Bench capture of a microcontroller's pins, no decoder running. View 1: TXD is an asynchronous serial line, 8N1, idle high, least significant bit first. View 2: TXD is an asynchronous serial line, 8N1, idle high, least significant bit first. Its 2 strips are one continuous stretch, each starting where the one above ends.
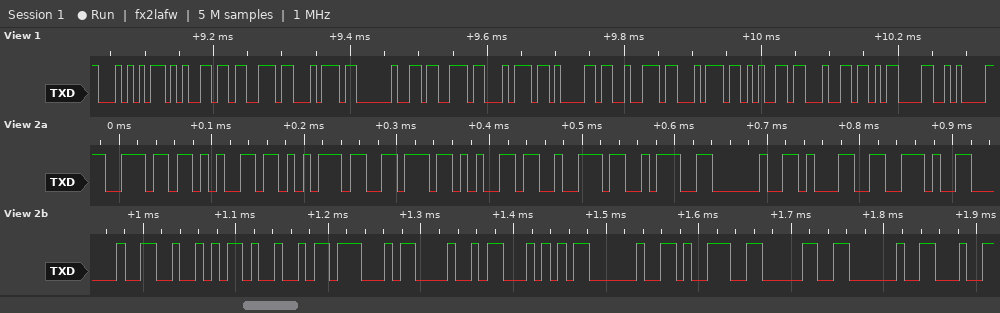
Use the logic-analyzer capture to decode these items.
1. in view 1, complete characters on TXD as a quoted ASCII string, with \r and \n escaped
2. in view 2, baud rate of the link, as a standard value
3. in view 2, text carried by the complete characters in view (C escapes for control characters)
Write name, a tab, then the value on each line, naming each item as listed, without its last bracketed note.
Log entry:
in view 1, complete characters on TXD as a quoted ASCII string, with \r and \n escaped	"Test started\r\n"
in view 2, baud rate of the link, as a standard value	115200 baud
in view 2, text carried by the complete characters in view	"neuver: 1. RIGHT 90 "
